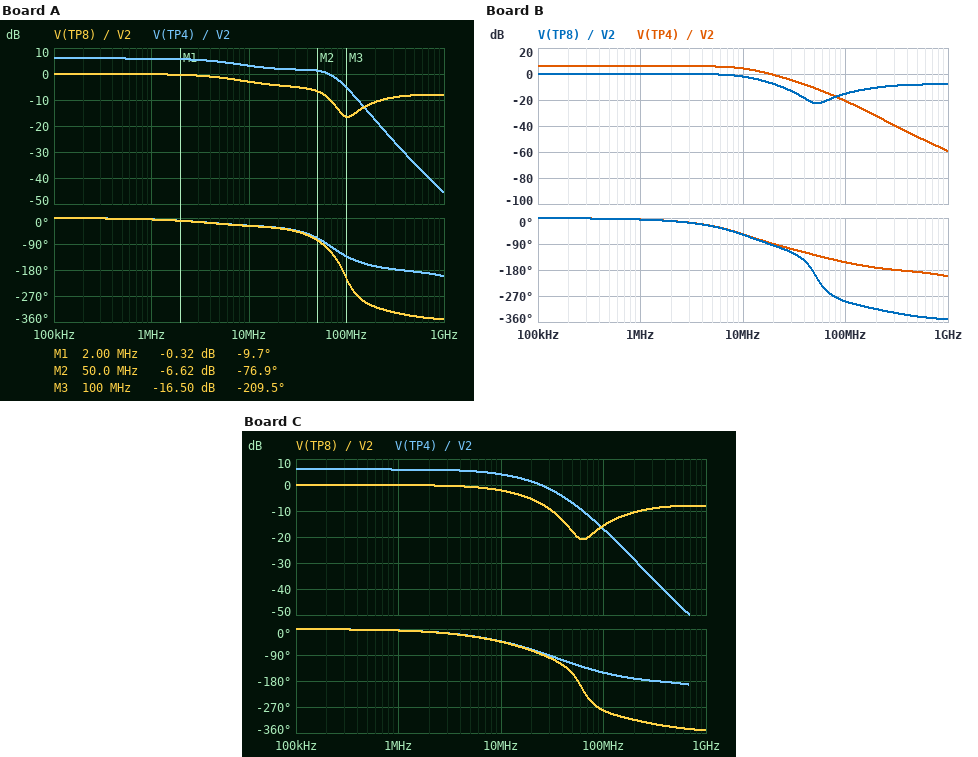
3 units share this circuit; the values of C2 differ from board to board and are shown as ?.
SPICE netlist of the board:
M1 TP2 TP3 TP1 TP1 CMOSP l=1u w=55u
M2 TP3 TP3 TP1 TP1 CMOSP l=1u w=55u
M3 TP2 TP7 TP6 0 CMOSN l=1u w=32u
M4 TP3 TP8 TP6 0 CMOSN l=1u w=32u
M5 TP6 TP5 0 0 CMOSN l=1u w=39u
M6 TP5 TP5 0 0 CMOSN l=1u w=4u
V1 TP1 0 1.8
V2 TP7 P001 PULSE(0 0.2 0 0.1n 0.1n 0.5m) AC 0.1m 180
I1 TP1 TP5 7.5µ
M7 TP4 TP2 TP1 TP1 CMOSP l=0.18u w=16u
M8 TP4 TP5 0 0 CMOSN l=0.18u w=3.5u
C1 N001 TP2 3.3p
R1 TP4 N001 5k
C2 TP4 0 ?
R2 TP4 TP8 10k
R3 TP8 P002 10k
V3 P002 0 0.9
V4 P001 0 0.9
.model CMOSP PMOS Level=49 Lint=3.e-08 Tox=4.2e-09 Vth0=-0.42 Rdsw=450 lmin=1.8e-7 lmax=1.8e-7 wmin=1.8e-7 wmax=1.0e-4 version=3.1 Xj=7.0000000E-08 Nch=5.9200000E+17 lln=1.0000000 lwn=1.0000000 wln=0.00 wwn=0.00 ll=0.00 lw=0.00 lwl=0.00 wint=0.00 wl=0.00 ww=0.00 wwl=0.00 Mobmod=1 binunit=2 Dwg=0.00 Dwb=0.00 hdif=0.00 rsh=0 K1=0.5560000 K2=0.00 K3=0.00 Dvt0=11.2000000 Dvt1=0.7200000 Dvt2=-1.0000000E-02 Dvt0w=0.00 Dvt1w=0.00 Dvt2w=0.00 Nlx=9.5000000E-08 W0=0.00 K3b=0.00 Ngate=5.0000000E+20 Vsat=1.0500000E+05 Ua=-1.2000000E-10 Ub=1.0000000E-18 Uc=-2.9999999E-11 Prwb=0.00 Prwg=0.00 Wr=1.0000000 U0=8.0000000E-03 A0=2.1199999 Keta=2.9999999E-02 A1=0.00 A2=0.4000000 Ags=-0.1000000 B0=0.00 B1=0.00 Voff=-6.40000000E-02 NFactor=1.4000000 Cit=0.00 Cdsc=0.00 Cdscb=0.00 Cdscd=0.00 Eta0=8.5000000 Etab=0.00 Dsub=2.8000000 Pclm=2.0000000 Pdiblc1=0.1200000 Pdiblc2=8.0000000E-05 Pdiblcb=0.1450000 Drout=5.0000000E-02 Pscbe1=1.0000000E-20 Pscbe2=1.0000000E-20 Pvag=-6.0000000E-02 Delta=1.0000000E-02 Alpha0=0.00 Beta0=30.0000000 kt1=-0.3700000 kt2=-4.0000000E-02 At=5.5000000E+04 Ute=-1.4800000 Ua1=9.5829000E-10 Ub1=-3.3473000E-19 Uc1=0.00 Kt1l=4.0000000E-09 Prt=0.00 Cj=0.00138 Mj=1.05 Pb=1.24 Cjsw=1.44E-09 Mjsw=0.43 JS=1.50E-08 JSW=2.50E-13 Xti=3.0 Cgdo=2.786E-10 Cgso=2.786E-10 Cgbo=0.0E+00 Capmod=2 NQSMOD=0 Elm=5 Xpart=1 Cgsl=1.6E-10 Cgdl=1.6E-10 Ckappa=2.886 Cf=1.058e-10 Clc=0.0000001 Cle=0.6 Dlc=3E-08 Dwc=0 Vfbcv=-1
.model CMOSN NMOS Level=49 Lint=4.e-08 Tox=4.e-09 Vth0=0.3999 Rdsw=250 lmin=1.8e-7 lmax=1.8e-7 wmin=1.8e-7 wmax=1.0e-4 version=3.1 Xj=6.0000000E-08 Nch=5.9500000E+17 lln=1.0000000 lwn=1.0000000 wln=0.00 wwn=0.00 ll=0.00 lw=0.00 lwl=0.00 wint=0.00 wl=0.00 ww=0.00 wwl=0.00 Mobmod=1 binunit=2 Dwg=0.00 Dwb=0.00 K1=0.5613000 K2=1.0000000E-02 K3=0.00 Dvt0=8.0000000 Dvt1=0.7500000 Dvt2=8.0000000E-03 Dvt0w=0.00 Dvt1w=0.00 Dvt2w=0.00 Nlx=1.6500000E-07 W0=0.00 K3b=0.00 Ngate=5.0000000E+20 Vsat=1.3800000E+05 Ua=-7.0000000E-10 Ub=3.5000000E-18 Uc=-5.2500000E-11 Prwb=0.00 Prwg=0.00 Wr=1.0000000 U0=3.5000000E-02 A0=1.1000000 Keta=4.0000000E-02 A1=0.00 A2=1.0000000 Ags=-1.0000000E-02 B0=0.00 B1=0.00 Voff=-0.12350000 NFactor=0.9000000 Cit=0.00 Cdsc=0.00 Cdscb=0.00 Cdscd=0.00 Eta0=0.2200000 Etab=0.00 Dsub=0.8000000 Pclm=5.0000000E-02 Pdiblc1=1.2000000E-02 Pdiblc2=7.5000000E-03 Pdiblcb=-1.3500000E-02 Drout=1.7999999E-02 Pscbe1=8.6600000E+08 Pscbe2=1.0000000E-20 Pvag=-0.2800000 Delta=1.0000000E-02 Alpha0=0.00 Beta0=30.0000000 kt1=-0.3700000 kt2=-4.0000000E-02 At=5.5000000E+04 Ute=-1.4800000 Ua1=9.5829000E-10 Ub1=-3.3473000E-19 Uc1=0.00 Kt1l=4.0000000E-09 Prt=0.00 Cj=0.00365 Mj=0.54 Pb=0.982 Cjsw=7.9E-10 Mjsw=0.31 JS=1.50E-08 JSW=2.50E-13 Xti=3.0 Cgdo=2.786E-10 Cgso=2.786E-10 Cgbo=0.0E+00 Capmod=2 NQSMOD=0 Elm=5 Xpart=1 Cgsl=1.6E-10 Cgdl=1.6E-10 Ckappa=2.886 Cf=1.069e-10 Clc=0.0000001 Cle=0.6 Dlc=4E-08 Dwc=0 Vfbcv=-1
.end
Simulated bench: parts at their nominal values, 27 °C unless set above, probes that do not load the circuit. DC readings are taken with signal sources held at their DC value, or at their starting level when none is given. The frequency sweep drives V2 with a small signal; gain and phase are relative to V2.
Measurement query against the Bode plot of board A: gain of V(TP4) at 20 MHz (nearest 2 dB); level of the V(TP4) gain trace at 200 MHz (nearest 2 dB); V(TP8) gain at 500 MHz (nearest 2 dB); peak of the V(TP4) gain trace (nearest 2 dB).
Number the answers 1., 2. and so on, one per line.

1. 2 dB
2. -18 dB
3. -8 dB
4. 6 dB
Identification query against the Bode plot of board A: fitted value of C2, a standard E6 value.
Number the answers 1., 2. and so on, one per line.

1. 6.8 pF
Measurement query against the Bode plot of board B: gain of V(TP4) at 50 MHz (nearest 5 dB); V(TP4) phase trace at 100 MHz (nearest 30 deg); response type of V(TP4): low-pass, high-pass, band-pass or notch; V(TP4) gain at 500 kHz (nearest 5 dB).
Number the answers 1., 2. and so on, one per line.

1. -10 dB
2. -150 deg
3. low-pass
4. 5 dB
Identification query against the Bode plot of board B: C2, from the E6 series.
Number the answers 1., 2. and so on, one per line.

1. 33 pF
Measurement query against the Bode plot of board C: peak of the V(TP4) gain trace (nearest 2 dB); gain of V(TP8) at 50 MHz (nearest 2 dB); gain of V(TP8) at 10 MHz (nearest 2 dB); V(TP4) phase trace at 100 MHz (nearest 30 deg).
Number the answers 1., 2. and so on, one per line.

1. 6 dB
2. -18 dB
3. -2 dB
4. -150 deg
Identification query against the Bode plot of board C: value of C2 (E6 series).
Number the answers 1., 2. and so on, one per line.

1. 22 pF
